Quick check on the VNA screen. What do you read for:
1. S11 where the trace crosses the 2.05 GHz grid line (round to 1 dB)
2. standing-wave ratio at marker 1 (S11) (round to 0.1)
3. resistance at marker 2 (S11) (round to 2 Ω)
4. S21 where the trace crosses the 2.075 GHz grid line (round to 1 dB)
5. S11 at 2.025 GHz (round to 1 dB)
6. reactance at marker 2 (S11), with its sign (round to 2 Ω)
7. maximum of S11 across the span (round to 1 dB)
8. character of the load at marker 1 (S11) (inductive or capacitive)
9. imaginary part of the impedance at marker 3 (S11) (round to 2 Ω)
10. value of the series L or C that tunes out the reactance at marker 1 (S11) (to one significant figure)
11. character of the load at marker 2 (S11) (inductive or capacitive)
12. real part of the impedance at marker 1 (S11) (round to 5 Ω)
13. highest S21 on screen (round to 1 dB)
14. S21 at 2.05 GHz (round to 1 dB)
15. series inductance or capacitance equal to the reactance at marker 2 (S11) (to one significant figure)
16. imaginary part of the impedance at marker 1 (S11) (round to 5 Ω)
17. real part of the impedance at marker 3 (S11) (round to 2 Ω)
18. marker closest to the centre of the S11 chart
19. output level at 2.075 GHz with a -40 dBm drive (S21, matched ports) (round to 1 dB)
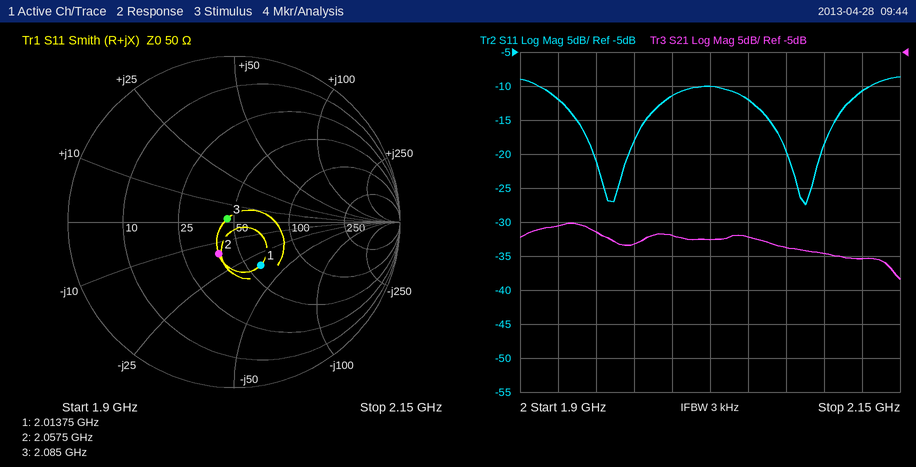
-12 dB
1.9
38 Ω
-34 dB
-10 dB
-16 Ω
-9 dB
capacitive
+2 Ω
3 nH
capacitive
60 Ω
-30 dB
-32 dB
5 pF
-35 Ω
46 Ω
marker 3
-74 dBm
